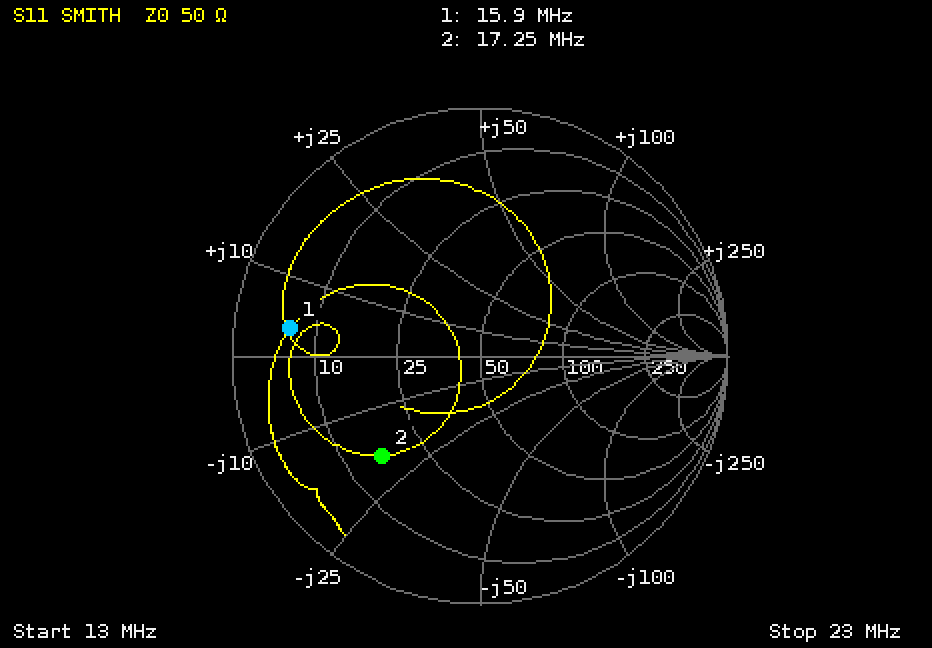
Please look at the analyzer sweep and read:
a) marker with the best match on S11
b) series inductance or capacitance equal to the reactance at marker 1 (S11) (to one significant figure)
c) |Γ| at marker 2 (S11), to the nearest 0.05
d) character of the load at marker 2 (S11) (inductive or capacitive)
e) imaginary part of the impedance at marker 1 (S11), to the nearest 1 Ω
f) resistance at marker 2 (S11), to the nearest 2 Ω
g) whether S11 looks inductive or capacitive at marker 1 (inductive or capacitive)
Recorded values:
marker 2
40 nH
0.55
capacitive
+4 Ω
16 Ω
inductive
